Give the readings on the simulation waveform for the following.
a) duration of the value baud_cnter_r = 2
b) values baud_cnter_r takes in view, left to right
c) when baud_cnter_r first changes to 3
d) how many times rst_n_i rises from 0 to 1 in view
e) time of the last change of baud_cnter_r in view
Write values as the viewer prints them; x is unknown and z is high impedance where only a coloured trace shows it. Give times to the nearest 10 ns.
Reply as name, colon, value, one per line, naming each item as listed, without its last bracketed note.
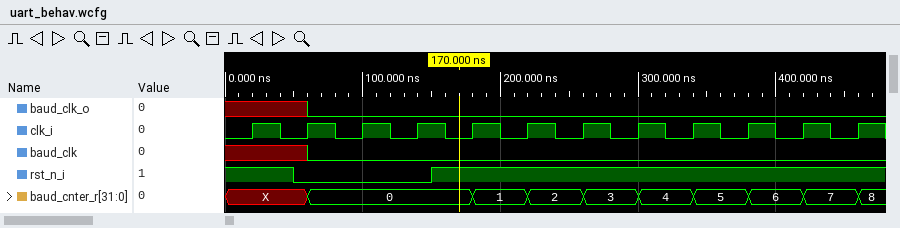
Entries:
duration of the value baud_cnter_r = 2: 40 ns
values baud_cnter_r takes in view, left to right: X, 0, 1, 2, 3, 4, 5, 6, 7, 8
when baud_cnter_r first changes to 3: 260 ns
how many times rst_n_i rises from 0 to 1 in view: 1
time of the last change of baud_cnter_r in view: 460 ns
